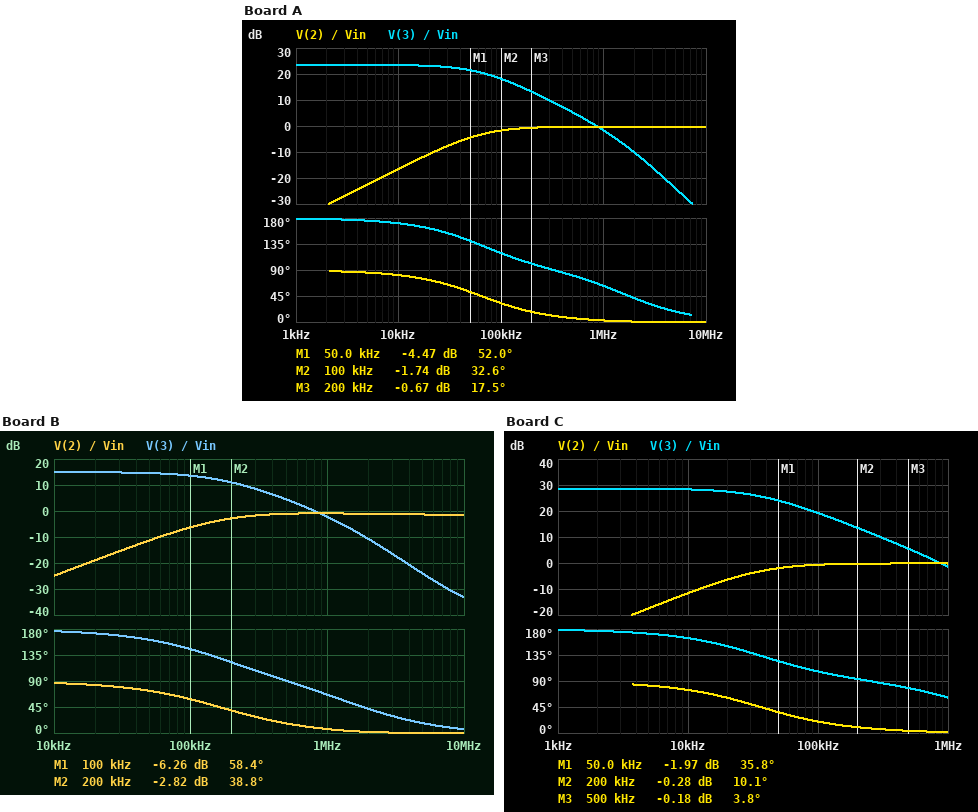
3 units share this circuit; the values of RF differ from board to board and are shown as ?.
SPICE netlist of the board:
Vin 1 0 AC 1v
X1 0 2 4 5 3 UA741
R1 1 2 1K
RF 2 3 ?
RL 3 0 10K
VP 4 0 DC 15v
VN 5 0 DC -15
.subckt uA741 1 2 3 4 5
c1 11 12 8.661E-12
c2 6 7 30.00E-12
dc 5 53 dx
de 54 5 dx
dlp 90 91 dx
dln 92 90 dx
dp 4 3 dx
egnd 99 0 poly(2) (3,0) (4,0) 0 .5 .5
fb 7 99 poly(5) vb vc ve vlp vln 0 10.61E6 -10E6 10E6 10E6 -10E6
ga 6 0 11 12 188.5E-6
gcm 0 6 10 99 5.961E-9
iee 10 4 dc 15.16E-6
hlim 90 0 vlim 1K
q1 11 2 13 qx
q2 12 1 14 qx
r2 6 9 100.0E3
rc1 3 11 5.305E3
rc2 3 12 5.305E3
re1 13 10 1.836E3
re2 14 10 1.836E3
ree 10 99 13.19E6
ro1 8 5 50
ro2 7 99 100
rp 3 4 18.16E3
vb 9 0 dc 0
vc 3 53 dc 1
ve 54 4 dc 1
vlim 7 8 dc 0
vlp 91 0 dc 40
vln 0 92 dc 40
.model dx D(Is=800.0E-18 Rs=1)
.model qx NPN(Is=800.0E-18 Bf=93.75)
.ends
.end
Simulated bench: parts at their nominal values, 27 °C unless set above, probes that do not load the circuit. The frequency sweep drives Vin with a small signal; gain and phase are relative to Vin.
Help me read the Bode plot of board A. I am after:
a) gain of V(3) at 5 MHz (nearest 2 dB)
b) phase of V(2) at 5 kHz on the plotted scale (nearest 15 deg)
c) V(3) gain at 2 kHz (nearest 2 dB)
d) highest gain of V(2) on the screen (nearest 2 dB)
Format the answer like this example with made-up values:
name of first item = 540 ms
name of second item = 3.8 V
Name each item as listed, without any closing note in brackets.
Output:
gain of V(3) at 5 MHz = -24 dB
phase of V(2) at 5 kHz on the plotted scale = 90 deg
V(3) gain at 2 kHz = 24 dB
highest gain of V(2) on the screen = 0 dB
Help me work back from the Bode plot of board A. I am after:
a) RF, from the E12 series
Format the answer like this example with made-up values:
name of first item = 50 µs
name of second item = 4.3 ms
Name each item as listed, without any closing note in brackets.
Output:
RF, from the E12 series = 15 kΩ
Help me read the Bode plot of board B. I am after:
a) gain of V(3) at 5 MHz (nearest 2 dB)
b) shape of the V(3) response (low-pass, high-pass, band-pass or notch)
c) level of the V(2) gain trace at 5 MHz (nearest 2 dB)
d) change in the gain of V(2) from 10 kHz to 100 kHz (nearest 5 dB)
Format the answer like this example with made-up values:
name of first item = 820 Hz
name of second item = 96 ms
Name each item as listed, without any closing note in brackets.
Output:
gain of V(3) at 5 MHz = -24 dB
shape of the V(3) response = low-pass
level of the V(2) gain trace at 5 MHz = -2 dB
change in the gain of V(2) from 10 kHz to 100 kHz = 20 dB
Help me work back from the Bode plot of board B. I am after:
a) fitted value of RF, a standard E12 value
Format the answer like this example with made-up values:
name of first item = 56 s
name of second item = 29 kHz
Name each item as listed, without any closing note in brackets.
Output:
fitted value of RF, a standard E12 value = 5.6 kΩ
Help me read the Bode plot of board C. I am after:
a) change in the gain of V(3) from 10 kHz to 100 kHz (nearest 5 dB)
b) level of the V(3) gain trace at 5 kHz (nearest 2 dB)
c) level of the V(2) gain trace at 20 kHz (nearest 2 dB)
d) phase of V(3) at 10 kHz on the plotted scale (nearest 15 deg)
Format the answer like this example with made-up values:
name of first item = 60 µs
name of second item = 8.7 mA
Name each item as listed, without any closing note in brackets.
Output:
change in the gain of V(3) from 10 kHz to 100 kHz = -10 dB
level of the V(3) gain trace at 5 kHz = 28 dB
level of the V(2) gain trace at 20 kHz = -6 dB
phase of V(3) at 10 kHz on the plotted scale = 165 deg
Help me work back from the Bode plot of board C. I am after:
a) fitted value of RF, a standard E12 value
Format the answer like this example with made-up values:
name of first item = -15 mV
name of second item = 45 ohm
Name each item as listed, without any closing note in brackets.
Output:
fitted value of RF, a standard E12 value = 27 kΩ
